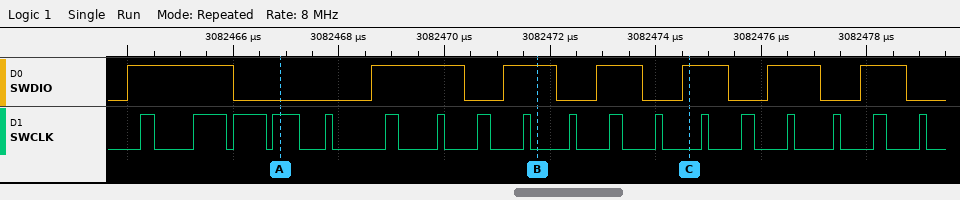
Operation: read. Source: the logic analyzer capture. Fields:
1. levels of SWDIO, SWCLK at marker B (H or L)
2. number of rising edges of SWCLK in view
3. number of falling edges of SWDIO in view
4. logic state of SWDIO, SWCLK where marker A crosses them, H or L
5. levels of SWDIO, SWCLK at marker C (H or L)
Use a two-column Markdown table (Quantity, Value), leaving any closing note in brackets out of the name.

| Quantity | Value |
|---|---|
| levels of SWDIO, SWCLK at marker B | SWDIO=H, SWCLK=L |
| number of rising edges of SWCLK in view | 18 |
| number of falling edges of SWDIO in view | 7 |
| logic state of SWDIO, SWCLK where marker A crosses them, H or L | SWDIO=L, SWCLK=H |
| levels of SWDIO, SWCLK at marker C | SWDIO=H, SWCLK=L |
